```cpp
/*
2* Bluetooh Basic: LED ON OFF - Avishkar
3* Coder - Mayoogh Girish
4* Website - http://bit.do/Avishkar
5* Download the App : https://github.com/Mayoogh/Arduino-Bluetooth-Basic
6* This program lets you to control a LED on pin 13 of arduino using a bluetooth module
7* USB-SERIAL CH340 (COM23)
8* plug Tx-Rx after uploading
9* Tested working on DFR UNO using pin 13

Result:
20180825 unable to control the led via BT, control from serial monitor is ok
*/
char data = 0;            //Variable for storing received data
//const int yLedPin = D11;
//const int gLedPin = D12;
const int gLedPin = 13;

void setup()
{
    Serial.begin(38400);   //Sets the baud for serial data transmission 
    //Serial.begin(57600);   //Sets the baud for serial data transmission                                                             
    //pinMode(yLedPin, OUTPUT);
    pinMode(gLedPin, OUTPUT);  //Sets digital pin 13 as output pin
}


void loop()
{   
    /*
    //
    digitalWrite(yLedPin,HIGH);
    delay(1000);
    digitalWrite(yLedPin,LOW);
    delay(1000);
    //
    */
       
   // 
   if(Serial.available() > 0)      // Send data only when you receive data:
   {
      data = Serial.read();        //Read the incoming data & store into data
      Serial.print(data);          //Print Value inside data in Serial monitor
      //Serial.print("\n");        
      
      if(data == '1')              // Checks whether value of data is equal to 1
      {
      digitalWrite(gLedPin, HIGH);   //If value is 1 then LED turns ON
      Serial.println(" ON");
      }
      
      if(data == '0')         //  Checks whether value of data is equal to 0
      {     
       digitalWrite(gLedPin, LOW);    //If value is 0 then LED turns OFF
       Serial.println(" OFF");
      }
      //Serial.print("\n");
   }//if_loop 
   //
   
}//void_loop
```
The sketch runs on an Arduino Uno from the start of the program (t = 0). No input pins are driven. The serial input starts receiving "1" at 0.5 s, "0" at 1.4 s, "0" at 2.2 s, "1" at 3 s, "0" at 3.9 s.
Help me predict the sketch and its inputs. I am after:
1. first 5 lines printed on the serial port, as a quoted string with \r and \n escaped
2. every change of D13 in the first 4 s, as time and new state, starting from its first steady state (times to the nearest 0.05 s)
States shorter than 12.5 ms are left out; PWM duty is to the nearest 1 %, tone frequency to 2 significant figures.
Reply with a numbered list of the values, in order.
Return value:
1. "1 ON\r\n0 OFF\r\n0 OFF\r\n1 ON\r\n0 OFF\r\n"
2. 0 s low; 0.5 s high; 1.4 s low; 3 s high; 3.9 s low
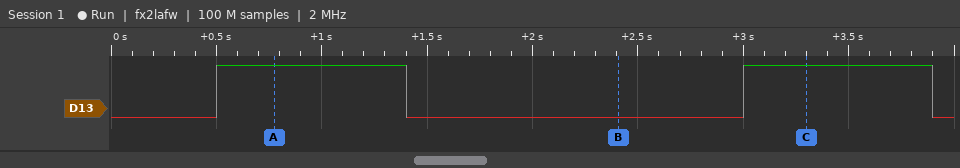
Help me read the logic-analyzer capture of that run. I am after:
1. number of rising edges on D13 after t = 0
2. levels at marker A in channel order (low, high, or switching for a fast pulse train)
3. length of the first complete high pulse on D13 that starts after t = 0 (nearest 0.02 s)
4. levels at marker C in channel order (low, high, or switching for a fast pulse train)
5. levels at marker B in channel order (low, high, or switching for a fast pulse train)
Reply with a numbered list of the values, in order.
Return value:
1. 2
2. D13 high
3. 0.90 s
4. D13 high
5. D13 low
